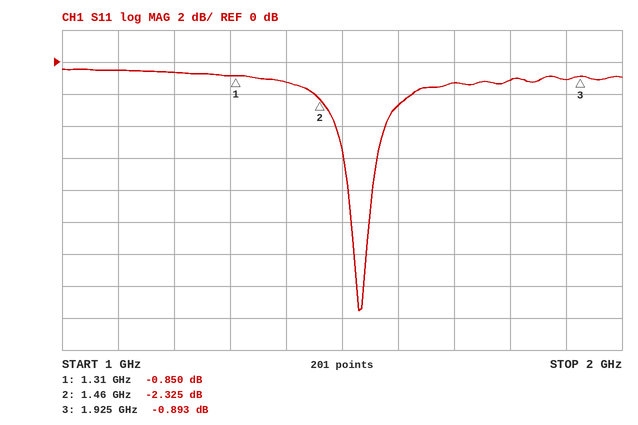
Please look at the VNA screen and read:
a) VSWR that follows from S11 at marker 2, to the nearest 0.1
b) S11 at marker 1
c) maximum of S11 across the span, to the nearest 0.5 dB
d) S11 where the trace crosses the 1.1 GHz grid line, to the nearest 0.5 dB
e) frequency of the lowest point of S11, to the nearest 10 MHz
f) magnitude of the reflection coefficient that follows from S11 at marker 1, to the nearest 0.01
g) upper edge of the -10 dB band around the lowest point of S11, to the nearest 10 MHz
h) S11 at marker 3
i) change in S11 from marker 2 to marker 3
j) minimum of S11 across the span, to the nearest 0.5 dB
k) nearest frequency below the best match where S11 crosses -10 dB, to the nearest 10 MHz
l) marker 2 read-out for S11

7.5
-0.850 dB
-0.5 dB
-0.5 dB
1.53 GHz
0.91
1.55 GHz
-0.893 dB
1.432 dB
-15.5 dB
1.52 GHz
-2.325 dB
